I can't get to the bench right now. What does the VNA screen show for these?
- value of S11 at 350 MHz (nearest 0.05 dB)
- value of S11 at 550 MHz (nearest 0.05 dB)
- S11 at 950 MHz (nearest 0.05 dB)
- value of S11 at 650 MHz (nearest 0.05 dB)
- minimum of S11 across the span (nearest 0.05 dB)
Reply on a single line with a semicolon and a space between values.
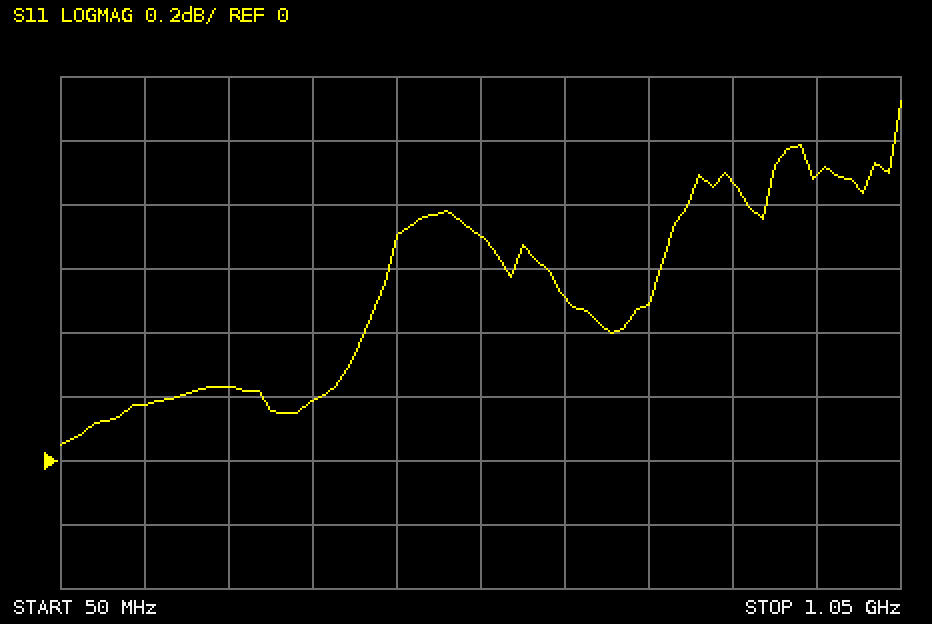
0.20 dB; 0.70 dB; 0.90 dB; 0.50 dB; 0.05 dB
